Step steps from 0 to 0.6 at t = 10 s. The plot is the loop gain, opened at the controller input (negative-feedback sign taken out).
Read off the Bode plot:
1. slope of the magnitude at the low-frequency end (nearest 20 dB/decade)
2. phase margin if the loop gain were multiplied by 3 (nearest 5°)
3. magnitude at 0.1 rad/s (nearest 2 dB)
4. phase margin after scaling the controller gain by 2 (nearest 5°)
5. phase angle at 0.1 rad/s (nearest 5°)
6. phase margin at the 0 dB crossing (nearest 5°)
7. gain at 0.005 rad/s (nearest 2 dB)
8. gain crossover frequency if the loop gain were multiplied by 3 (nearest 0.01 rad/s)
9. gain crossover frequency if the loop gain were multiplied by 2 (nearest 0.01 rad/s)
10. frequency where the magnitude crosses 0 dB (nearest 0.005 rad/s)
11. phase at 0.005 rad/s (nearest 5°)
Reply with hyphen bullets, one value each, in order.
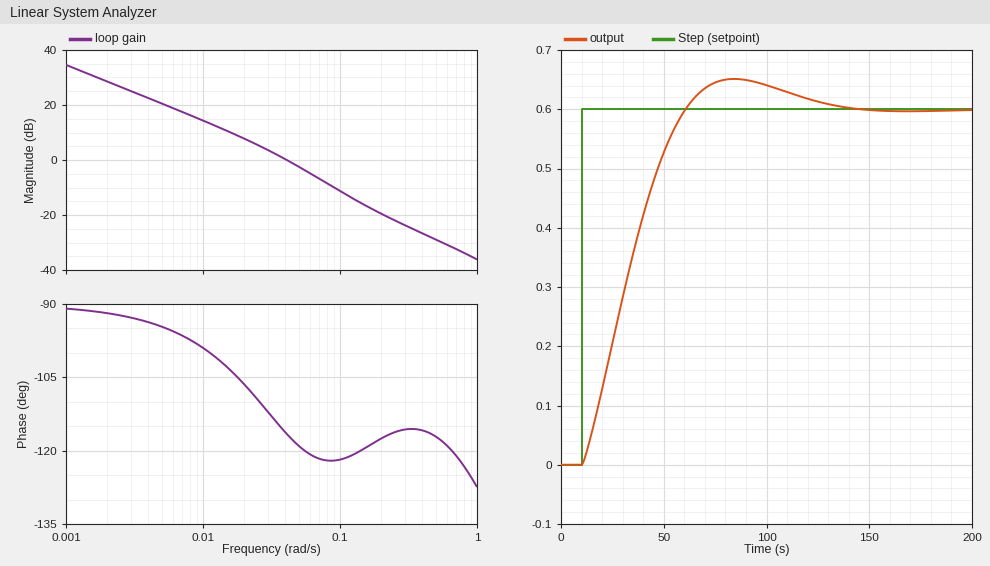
- -20 dB/decade
- 60°
- -12 dB
- 60°
- -120°
- 65°
- 20 dB
- 0.09 rad/s
- 0.07 rad/s
- 0.040 rad/s
- -95°
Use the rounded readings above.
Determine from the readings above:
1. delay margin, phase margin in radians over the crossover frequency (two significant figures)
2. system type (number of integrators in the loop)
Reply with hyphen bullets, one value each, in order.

- 28 s
- 1
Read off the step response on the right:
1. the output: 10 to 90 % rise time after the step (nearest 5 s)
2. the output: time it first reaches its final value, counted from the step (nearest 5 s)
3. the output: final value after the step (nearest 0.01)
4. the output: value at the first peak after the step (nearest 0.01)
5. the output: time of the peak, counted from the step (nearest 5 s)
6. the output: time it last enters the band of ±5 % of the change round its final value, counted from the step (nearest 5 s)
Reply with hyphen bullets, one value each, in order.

- 35 s
- 50 s
- 0.60
- 0.65
- 75 s
- 100 s
